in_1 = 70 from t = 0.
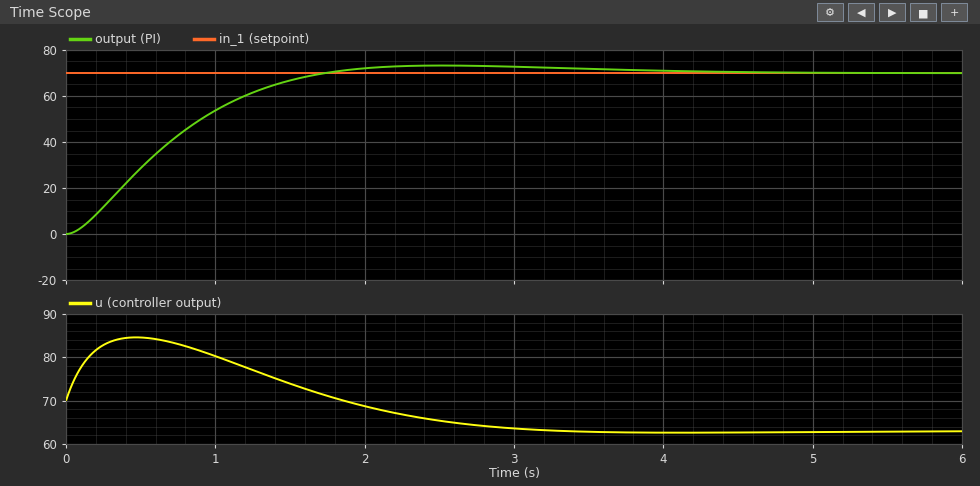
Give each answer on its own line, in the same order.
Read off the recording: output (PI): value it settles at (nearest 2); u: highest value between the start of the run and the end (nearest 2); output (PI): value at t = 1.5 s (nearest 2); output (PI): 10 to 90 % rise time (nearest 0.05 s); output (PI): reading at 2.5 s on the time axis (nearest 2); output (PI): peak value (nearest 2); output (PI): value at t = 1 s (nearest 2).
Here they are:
70
84
66
1.15 s
74
74
54
